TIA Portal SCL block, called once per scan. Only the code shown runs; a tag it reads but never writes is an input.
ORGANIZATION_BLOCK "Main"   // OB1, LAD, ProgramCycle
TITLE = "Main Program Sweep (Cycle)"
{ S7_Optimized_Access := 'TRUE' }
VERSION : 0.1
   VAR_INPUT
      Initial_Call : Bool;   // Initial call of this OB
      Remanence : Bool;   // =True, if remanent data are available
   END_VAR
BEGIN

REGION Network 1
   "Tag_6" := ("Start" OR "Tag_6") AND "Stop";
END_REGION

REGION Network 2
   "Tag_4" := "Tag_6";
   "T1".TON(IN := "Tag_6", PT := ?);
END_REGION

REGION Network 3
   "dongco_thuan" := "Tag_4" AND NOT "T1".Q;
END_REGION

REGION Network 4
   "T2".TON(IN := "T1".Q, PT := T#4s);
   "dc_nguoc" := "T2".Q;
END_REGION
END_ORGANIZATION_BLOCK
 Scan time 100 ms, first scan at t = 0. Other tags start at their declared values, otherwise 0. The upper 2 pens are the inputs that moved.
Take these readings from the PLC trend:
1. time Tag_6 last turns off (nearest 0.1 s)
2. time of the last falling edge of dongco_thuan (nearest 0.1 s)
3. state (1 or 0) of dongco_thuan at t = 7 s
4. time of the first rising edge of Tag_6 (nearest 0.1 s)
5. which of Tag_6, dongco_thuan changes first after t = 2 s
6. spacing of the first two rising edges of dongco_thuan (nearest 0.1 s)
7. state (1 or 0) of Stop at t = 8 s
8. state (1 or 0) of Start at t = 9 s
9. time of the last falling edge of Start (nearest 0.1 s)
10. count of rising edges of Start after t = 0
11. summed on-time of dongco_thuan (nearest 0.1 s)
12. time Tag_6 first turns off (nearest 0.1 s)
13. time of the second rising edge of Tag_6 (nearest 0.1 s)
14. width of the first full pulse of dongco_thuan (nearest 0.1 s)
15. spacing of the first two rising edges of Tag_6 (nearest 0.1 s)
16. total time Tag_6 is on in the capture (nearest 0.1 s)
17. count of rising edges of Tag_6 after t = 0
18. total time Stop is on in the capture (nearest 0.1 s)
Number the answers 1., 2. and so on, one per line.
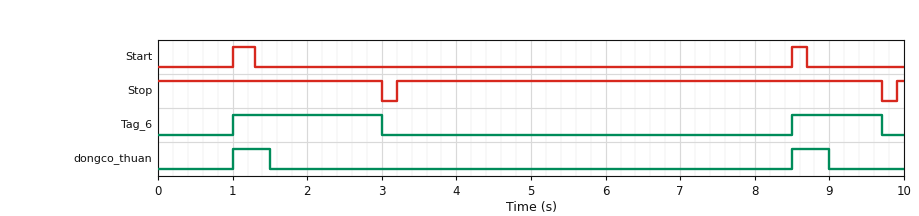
1. 9.7 s
2. 9.0 s
3. 0
4. 1.0 s
5. Tag_6
6. 7.5 s
7. 1
8. 0
9. 8.7 s
10. 2
11. 1.0 s
12. 3.0 s
13. 8.5 s
14. 0.5 s
15. 7.5 s
16. 3.2 s
17. 2
18. 9.6 s
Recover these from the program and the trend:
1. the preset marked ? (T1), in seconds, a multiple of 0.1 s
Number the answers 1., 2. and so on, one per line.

1. 0.5 s
